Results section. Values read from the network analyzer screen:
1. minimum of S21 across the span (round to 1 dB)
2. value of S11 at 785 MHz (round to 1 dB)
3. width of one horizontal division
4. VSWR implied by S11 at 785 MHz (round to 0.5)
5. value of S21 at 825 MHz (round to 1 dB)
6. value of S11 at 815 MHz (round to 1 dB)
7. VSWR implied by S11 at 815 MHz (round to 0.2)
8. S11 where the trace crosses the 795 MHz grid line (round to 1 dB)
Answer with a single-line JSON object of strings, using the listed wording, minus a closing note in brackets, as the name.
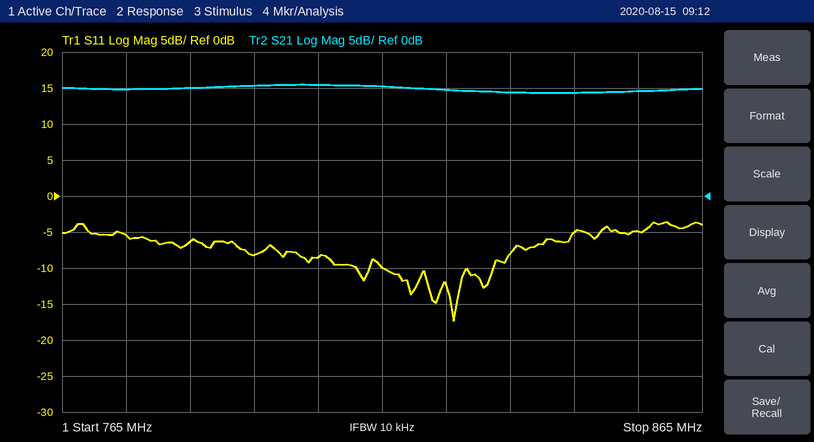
{"minimum of S21 across the span": "14 dB", "value of S11 at 785 MHz": "-6 dB", "width of one horizontal division": "10 MHz", "VSWR implied by S11 at 785 MHz": "3.0", "value of S21 at 825 MHz": "15 dB", "value of S11 at 815 MHz": "-10 dB", "VSWR implied by S11 at 815 MHz": "2.0", "S11 where the trace crosses the 795 MHz grid line": "-8 dB"}
